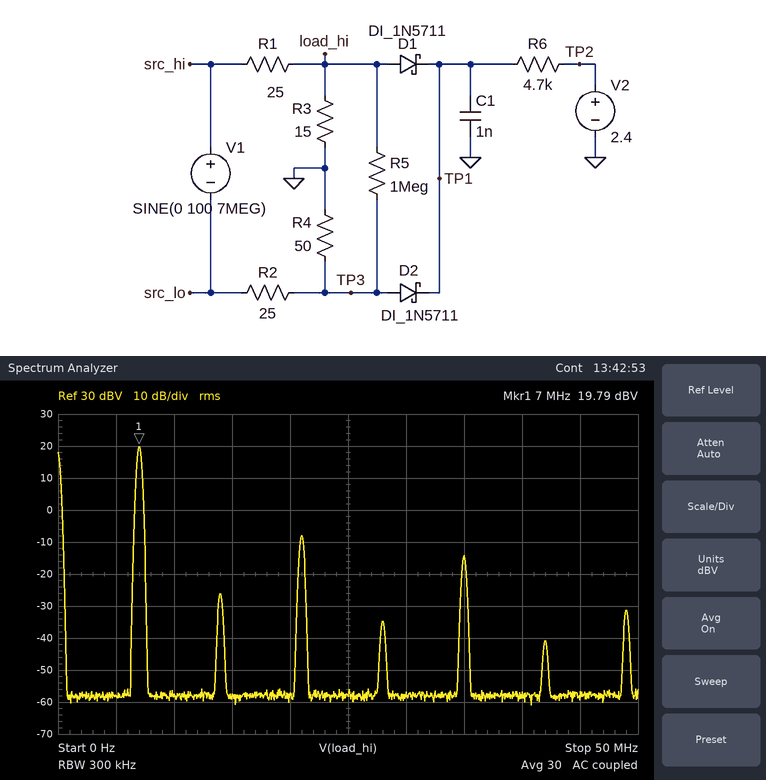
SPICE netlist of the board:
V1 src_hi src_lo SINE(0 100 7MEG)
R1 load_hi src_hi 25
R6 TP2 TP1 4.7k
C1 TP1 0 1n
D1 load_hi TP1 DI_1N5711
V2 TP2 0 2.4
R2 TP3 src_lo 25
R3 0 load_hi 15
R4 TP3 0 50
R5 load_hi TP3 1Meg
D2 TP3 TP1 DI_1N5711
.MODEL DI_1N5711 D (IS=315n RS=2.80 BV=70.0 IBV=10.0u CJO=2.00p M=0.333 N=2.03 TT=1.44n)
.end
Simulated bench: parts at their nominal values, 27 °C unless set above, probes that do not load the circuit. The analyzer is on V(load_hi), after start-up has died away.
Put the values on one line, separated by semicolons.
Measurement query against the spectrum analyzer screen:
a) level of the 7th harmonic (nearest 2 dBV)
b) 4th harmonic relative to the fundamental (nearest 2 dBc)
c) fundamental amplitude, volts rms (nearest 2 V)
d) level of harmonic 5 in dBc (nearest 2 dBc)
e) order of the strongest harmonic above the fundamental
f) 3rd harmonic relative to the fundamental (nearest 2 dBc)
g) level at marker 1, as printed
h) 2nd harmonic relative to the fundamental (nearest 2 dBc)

-32 dBV; -54 dBc; 10 V; -34 dBc; 3; -28 dBc; 19.79 dBV; -46 dBc
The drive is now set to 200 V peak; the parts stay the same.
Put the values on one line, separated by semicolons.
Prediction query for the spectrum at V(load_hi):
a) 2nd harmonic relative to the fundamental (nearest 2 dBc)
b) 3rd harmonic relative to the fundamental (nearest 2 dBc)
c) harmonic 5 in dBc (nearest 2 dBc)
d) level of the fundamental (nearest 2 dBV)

-52 dBc; -18 dBc; -28 dBc; 26 dBV
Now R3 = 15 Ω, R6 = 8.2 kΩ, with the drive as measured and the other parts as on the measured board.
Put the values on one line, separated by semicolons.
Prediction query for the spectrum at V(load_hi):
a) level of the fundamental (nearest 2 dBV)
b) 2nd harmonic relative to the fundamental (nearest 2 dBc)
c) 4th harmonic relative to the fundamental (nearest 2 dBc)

20 dBV; -50 dBc; -60 dBc
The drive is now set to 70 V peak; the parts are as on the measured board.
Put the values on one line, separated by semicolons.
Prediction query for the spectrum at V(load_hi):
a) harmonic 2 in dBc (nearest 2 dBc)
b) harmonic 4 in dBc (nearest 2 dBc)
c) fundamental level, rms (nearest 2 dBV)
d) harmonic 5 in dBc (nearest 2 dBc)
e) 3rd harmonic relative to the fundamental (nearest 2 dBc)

-42 dBc; -44 dBc; 16 dBV; -46 dBc; -44 dBc
